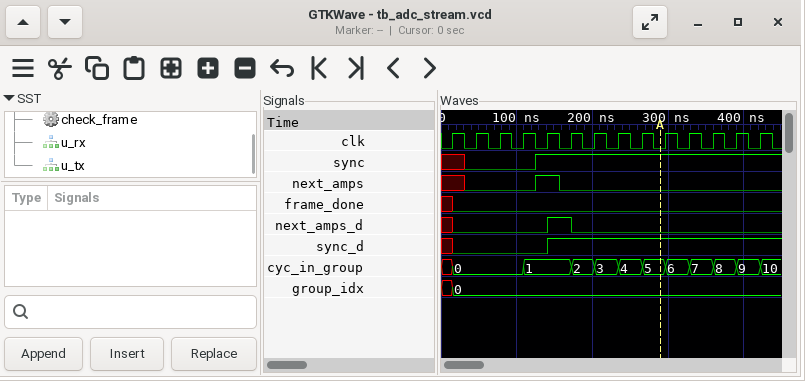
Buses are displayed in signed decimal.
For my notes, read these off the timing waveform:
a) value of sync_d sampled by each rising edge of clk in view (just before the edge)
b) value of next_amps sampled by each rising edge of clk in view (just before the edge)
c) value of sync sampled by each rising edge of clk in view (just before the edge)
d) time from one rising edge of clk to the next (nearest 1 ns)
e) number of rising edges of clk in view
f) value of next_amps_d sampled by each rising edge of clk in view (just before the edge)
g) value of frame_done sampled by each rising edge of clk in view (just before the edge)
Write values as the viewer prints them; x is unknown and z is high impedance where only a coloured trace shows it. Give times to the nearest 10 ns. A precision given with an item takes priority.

x 0 0 0 0 1 1 1 1 1 1 1 1 1
x 0 0 0 1 0 0 0 0 0 0 0 0 0
x 0 0 0 1 1 1 1 1 1 1 1 1 1
31 ns
14
x 0 0 0 0 1 0 0 0 0 0 0 0 0
x 0 0 0 0 0 0 0 0 0 0 0 0 0
